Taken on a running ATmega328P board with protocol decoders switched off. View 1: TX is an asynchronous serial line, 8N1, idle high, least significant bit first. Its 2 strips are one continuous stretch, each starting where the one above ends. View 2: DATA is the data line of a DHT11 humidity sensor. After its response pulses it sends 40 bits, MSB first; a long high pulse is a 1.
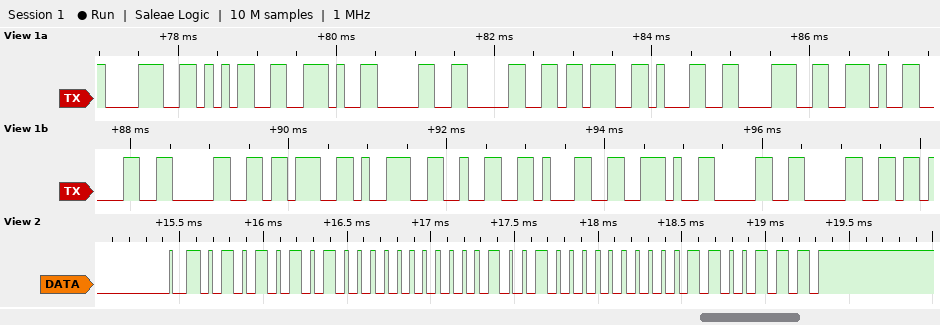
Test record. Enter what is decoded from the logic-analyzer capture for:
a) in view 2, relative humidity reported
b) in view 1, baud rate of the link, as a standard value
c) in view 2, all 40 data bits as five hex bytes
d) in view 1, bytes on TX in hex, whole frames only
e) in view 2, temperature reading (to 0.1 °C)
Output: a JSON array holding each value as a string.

["85 %", "9600 baud", "55 00 12 00 67", "38 35 2E 30 30 3B 31 38 2E 30 30 3B 39 32 31 2E 30 30", "18.0 °C"]
